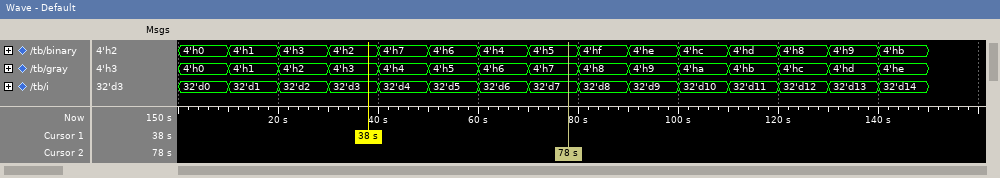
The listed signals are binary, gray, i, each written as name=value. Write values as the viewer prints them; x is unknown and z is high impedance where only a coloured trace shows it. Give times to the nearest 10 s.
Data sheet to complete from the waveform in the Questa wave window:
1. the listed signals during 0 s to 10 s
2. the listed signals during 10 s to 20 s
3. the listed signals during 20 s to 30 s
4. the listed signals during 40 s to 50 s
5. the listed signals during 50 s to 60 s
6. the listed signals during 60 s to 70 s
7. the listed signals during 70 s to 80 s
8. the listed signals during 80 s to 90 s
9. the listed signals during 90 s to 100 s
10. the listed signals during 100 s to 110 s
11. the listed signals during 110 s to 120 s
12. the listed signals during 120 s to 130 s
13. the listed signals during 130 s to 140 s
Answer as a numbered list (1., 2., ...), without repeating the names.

1. binary=4'h0, gray=4'h0, i=32'd0
2. binary=4'h1, gray=4'h1, i=32'd1
3. binary=4'h3, gray=4'h2, i=32'd2
4. binary=4'h7, gray=4'h4, i=32'd4
5. binary=4'h6, gray=4'h5, i=32'd5
6. binary=4'h4, gray=4'h6, i=32'd6
7. binary=4'h5, gray=4'h7, i=32'd7
8. binary=4'hf, gray=4'h8, i=32'd8
9. binary=4'he, gray=4'h9, i=32'd9
10. binary=4'hc, gray=4'ha, i=32'd10
11. binary=4'hd, gray=4'hb, i=32'd11
12. binary=4'h8, gray=4'hc, i=32'd12
13. binary=4'h9, gray=4'hd, i=32'd13
